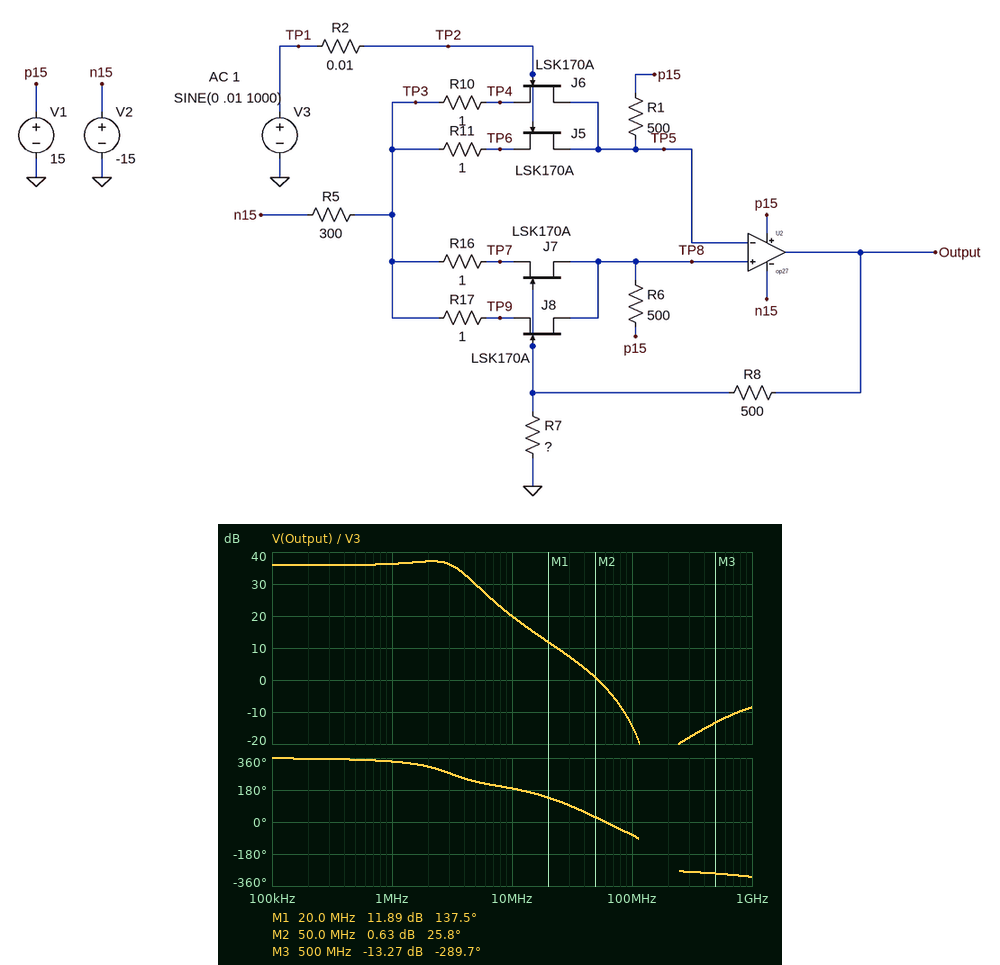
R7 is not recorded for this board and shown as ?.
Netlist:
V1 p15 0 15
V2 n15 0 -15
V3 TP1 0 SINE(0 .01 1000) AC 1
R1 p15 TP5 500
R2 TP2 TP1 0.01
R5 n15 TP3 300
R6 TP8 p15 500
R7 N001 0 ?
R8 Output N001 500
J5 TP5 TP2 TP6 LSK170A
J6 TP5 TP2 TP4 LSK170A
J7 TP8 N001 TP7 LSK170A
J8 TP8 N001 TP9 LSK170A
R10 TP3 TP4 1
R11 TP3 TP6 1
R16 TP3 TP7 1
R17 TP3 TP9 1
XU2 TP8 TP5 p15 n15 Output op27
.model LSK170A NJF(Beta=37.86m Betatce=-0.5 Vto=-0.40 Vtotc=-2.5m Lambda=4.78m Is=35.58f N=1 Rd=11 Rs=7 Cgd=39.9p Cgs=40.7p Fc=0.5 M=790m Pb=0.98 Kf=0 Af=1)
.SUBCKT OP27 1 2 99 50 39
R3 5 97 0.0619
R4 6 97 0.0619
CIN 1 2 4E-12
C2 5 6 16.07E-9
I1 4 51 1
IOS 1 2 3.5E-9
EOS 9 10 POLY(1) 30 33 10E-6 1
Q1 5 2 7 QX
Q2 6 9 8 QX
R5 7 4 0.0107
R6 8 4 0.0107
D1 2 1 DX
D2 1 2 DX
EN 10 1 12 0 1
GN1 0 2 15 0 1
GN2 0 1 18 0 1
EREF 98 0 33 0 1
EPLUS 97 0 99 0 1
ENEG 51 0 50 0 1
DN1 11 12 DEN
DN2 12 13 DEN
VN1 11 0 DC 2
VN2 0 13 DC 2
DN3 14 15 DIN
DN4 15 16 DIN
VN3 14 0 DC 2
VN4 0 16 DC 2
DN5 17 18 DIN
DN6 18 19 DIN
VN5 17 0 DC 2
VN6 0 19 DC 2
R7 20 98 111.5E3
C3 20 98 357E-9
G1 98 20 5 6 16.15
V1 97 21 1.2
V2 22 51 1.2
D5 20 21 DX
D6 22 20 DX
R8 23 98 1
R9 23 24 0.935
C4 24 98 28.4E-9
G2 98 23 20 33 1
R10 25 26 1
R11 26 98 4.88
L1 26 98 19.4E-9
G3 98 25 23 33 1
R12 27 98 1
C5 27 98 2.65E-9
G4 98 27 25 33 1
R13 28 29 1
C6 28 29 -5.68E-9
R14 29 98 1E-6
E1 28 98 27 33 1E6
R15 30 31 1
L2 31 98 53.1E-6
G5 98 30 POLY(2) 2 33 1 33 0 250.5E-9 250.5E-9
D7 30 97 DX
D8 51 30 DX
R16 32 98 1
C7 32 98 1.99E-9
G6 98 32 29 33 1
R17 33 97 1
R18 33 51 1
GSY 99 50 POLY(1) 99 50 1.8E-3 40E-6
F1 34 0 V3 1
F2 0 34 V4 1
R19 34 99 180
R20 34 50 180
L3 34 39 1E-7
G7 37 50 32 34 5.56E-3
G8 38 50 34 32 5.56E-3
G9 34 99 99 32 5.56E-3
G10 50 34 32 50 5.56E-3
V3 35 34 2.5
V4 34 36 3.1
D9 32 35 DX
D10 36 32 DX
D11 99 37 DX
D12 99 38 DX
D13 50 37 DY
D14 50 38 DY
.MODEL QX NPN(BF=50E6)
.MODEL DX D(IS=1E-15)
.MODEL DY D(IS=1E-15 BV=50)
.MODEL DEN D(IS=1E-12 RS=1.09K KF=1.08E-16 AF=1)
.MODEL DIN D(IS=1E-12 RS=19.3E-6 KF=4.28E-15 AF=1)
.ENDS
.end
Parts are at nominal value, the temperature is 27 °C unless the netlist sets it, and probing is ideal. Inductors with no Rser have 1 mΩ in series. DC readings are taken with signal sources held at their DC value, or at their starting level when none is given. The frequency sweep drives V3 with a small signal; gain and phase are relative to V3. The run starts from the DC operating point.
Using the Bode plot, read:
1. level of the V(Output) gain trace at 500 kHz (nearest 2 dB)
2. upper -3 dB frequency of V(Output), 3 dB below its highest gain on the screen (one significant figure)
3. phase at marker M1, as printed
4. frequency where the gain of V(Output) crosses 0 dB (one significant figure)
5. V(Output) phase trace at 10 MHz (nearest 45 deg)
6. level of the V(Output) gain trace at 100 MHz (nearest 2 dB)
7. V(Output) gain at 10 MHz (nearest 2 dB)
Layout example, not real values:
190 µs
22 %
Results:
36 dB
4 MHz
137.5 deg
50 MHz
180 deg
-14 dB
20 dB
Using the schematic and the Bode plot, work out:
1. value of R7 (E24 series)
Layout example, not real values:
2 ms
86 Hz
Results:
8.2 Ω
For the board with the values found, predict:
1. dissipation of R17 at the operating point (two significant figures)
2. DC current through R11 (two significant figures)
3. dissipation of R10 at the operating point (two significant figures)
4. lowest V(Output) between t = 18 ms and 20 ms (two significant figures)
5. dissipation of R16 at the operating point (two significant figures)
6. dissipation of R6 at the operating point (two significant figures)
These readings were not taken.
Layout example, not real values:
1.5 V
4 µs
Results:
150 µW
12 mA
150 µW
-620 mV
150 µW
300 mW
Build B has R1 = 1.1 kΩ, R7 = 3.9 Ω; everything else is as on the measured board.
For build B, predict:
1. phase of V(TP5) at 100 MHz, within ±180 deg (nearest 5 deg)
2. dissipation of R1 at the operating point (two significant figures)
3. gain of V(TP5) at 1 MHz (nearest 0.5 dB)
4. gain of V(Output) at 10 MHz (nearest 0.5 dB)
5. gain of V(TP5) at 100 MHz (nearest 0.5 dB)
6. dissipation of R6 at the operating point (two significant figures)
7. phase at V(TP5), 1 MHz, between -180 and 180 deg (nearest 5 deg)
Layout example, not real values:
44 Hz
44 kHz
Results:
15 deg
220 mW
-7.5 dB
-38.0 dB
-1.0 dB
460 mW
0 deg
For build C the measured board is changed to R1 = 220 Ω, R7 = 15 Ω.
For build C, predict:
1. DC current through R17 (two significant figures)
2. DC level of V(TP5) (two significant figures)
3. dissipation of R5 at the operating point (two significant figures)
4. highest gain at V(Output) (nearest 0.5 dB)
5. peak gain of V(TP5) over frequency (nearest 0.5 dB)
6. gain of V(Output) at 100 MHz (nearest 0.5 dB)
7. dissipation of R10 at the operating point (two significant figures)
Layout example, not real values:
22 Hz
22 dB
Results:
7.4 mA
7.6 V
710 mW
31.5 dB
18.5 dB
-13.0 dB
290 µW
